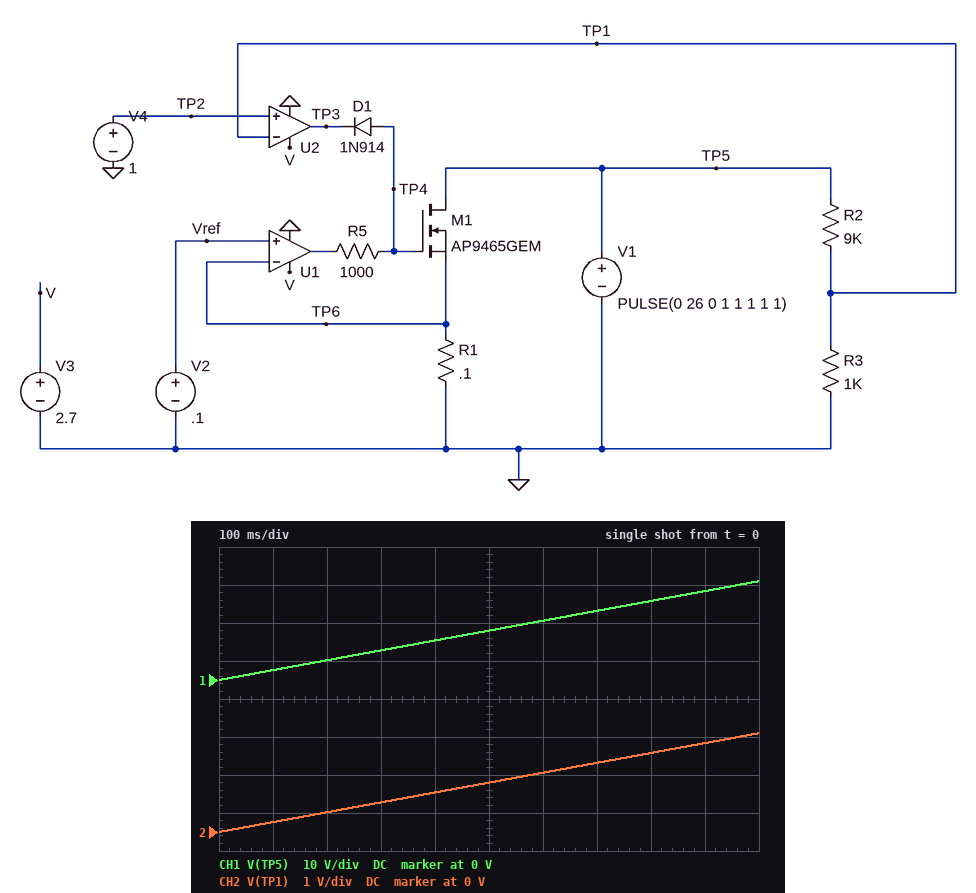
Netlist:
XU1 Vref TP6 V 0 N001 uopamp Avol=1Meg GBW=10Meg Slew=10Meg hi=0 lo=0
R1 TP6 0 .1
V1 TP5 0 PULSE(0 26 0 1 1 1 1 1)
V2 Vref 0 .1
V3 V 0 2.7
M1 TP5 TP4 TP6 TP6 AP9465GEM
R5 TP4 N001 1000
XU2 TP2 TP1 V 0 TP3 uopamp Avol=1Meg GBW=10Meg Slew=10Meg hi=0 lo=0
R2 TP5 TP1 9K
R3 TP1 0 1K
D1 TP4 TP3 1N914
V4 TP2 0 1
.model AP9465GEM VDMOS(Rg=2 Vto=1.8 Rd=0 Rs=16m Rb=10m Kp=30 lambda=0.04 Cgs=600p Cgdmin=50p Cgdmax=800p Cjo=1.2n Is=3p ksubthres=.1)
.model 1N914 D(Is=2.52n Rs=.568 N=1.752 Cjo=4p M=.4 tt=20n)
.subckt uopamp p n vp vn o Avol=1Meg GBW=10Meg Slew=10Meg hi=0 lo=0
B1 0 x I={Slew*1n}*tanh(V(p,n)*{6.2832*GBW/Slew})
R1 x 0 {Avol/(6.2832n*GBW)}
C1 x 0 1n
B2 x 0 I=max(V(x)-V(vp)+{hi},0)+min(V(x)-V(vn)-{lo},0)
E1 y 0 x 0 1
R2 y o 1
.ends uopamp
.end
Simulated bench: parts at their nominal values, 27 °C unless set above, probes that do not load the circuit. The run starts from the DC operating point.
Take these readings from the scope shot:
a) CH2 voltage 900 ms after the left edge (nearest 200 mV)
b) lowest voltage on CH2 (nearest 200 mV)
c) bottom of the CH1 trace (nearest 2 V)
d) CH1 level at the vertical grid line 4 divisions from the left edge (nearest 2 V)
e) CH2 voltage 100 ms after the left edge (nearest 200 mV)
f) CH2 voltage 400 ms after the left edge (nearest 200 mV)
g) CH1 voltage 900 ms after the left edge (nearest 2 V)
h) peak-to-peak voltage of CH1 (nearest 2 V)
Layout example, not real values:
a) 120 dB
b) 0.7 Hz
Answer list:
a) 2.4 V
b) 0 V
c) 0 V
d) 10 V
e) 200 mV
f) 1.0 V
g) 24 V
h) 26 V
